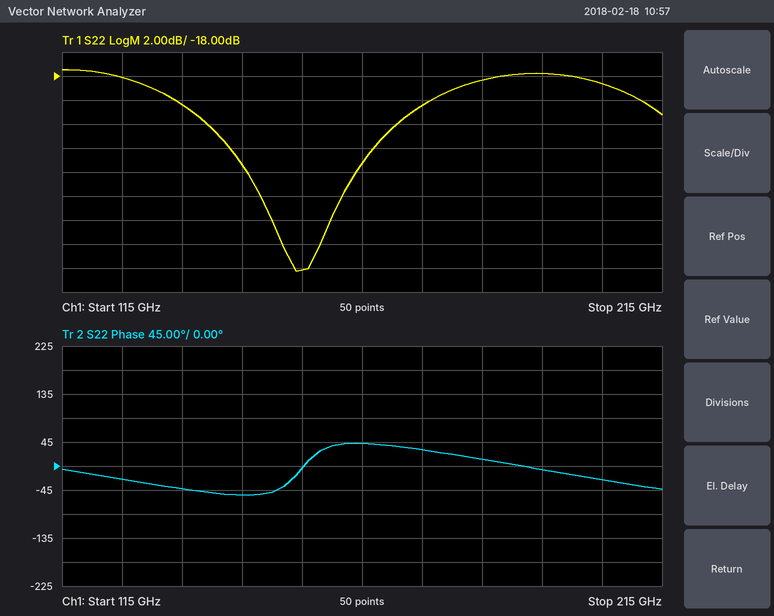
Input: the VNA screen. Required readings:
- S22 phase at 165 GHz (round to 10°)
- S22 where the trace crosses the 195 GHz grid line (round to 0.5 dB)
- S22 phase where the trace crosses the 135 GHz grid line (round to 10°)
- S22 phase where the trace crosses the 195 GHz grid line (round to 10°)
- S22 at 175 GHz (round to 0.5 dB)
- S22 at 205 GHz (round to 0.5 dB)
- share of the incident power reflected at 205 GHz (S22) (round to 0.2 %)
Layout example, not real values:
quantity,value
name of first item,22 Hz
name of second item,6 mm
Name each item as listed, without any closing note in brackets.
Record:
quantity,value
S22 phase at 165 GHz,40°
S22 where the trace crosses the 195 GHz grid line,-18.0 dB
S22 phase where the trace crosses the 135 GHz grid line,-40°
S22 phase where the trace crosses the 195 GHz grid line,-10°
S22 at 175 GHz,-20.5 dB
S22 at 205 GHz,-18.5 dB
share of the incident power reflected at 205 GHz (S22),1.4 %
